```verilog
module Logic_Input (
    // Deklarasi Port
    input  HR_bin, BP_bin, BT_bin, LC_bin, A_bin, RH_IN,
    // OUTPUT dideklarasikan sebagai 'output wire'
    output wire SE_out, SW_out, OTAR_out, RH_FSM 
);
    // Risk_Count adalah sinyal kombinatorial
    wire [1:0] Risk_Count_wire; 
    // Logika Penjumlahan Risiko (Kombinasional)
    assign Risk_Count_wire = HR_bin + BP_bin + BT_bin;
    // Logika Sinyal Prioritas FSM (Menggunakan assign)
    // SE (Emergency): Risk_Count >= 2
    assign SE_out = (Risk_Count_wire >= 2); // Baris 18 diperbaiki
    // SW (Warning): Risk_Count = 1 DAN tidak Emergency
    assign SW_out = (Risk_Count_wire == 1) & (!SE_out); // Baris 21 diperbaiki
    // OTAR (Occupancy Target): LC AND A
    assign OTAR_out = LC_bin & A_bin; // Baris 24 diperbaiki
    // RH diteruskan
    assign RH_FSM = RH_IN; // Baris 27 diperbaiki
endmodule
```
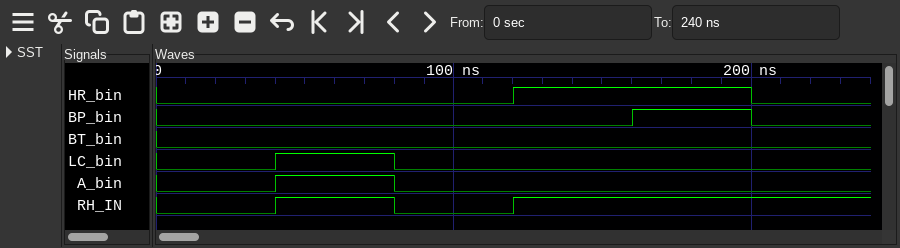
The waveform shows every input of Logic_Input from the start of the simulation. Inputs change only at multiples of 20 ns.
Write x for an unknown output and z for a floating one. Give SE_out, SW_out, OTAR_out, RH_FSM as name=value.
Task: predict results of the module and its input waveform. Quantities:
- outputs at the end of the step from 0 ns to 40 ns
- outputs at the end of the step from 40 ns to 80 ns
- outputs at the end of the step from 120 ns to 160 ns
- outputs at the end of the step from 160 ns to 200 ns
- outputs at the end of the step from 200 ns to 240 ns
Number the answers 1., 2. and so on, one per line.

1. SE_out=0, SW_out=0, OTAR_out=0, RH_FSM=0
2. SE_out=0, SW_out=0, OTAR_out=1, RH_FSM=1
3. SE_out=0, SW_out=1, OTAR_out=0, RH_FSM=1
4. SE_out=1, SW_out=0, OTAR_out=0, RH_FSM=1
5. SE_out=0, SW_out=0, OTAR_out=0, RH_FSM=1
